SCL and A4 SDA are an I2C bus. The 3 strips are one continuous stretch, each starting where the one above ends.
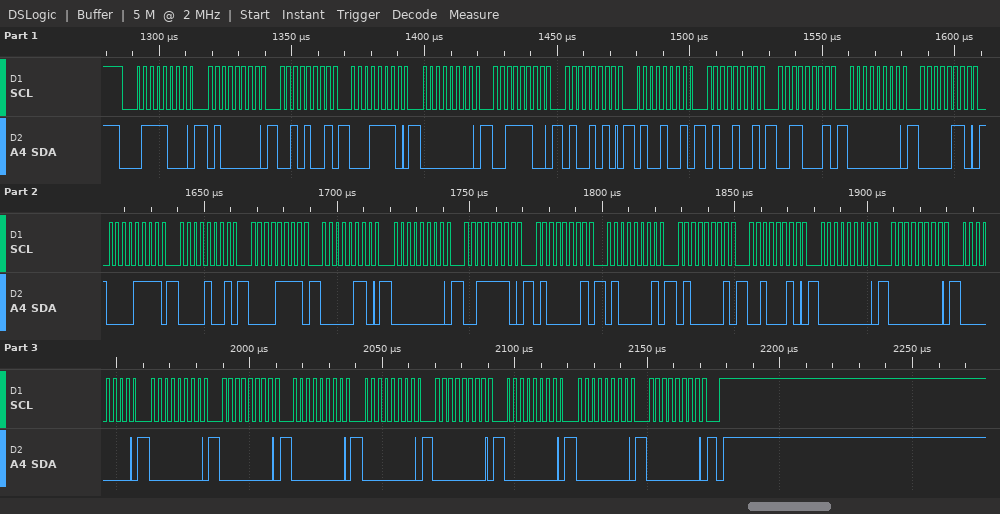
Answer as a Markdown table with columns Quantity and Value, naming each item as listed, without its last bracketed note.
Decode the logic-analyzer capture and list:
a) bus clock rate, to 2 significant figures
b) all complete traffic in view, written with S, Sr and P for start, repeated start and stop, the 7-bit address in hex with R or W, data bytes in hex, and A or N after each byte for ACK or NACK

| Quantity | Value |
|---|---|
| bus clock rate, to 2 significant figures | 400 kHz |
| all complete traffic in view, written with S, Sr and P for start, repeated start and stop, the 7-bit address in hex with R or W, data bytes in hex, and A or N after each byte for ACK or NACK | S 3CW A 40 A 29 A 1E A 00 A 3C A 4A A 49 A 49 A 31 A 00 A 06 A 0F A 09 A 0F A 06 A 00 A 3E A 41 A 41 A 41 A 22 A 00 A 00 A 00 A 00 A 00 A 00 A 00 A 00 A 00 A 00 A 00 A P |
